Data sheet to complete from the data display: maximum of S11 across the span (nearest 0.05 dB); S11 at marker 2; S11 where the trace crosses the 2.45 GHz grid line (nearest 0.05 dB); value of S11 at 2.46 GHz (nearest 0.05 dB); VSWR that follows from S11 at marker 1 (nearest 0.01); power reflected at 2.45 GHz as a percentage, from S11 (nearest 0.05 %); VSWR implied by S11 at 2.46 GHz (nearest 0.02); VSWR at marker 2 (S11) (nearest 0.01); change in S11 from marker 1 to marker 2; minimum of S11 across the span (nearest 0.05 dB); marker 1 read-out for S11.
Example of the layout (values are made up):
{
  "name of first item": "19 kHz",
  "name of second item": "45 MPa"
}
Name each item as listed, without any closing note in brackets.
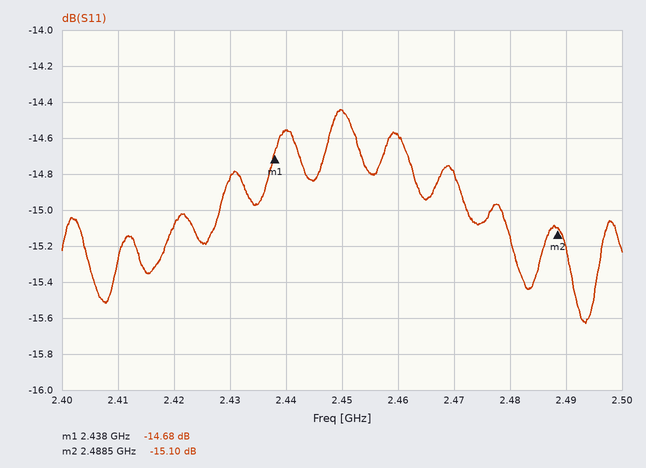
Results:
{
  "maximum of S11 across the span": "-14.45 dB",
  "S11 at marker 2": "-15.10 dB",
  "S11 where the trace crosses the 2.45 GHz grid line": "-14.45 dB",
  "value of S11 at 2.46 GHz": "-14.60 dB",
  "VSWR that follows from S11 at marker 1": "1.45",
  "power reflected at 2.45 GHz as a percentage, from S11": "3.60 %",
  "VSWR implied by S11 at 2.46 GHz": "1.46",
  "VSWR at marker 2 (S11)": "1.43",
  "change in S11 from marker 1 to marker 2": "-0.42 dB",
  "minimum of S11 across the span": "-15.65 dB",
  "marker 1 read-out for S11": "-14.68 dB"
}
